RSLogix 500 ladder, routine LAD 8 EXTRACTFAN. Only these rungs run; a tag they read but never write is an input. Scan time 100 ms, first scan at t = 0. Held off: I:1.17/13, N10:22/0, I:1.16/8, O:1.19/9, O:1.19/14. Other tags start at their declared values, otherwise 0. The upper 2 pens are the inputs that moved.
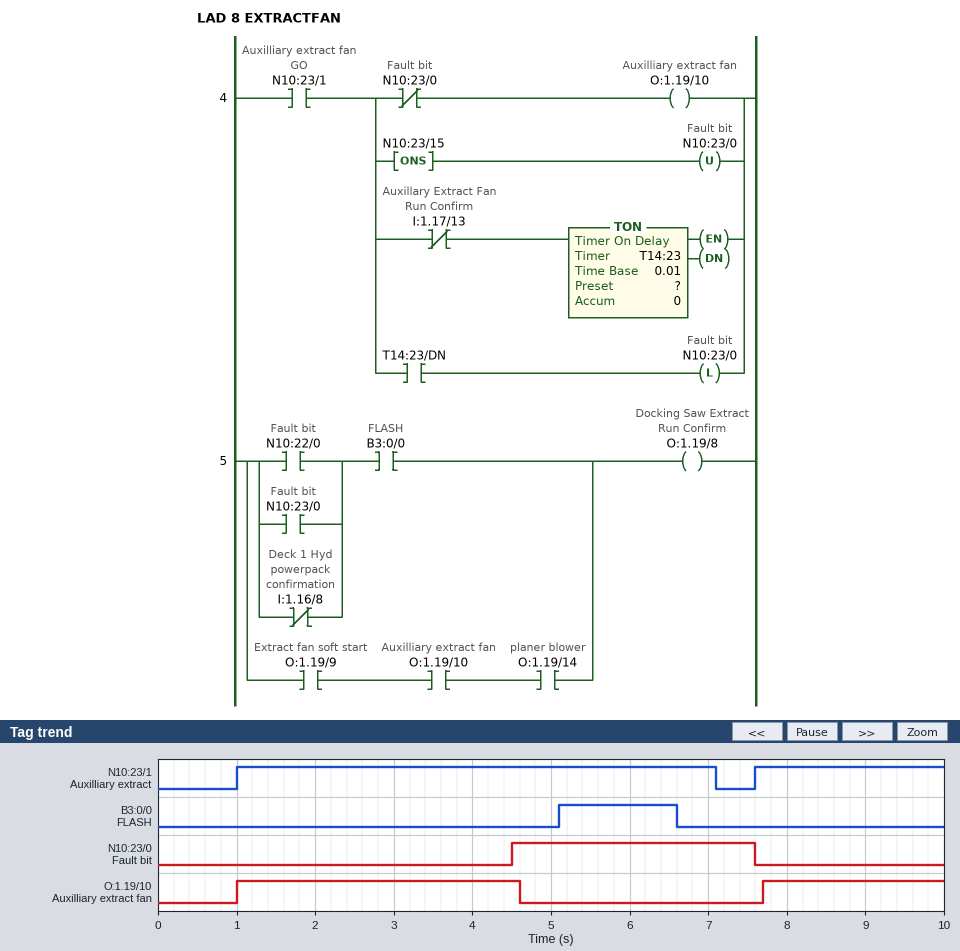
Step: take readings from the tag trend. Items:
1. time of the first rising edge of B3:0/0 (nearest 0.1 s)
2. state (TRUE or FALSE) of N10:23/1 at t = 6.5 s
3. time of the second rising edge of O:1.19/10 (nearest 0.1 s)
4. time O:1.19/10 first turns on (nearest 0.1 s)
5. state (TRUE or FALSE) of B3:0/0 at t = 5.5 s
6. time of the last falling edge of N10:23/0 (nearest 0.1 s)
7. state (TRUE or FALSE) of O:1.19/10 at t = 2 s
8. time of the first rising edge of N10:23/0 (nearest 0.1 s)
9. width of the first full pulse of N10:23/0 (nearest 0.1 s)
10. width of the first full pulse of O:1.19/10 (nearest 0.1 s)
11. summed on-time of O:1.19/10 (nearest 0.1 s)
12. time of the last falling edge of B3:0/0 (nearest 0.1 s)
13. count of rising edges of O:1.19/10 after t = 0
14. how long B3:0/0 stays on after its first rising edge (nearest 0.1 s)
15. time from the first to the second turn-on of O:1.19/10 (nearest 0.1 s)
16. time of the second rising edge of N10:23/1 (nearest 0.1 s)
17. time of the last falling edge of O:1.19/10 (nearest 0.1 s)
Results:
5.1 s
TRUE
7.7 s
1.0 s
TRUE
7.6 s
TRUE
4.5 s
3.1 s
3.6 s
5.9 s
6.6 s
2
1.5 s
6.7 s
7.6 s
4.6 s
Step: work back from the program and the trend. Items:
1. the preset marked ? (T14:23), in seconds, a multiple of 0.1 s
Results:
3.5 s
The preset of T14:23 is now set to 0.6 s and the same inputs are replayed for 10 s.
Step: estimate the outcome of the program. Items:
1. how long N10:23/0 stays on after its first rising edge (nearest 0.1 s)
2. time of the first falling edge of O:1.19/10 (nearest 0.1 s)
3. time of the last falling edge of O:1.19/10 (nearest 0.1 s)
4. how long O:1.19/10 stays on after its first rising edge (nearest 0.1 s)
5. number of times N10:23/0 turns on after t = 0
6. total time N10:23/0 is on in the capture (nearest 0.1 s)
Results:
6.0 s
1.7 s
8.3 s
0.7 s
2
7.8 s
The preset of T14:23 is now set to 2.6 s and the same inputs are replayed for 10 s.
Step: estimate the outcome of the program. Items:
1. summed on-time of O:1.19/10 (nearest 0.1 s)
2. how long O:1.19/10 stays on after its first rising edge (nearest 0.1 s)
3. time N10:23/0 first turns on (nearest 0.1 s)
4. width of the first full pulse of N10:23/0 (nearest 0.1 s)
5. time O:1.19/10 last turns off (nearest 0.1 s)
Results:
5.0 s
2.7 s
3.6 s
4.0 s
3.7 s
